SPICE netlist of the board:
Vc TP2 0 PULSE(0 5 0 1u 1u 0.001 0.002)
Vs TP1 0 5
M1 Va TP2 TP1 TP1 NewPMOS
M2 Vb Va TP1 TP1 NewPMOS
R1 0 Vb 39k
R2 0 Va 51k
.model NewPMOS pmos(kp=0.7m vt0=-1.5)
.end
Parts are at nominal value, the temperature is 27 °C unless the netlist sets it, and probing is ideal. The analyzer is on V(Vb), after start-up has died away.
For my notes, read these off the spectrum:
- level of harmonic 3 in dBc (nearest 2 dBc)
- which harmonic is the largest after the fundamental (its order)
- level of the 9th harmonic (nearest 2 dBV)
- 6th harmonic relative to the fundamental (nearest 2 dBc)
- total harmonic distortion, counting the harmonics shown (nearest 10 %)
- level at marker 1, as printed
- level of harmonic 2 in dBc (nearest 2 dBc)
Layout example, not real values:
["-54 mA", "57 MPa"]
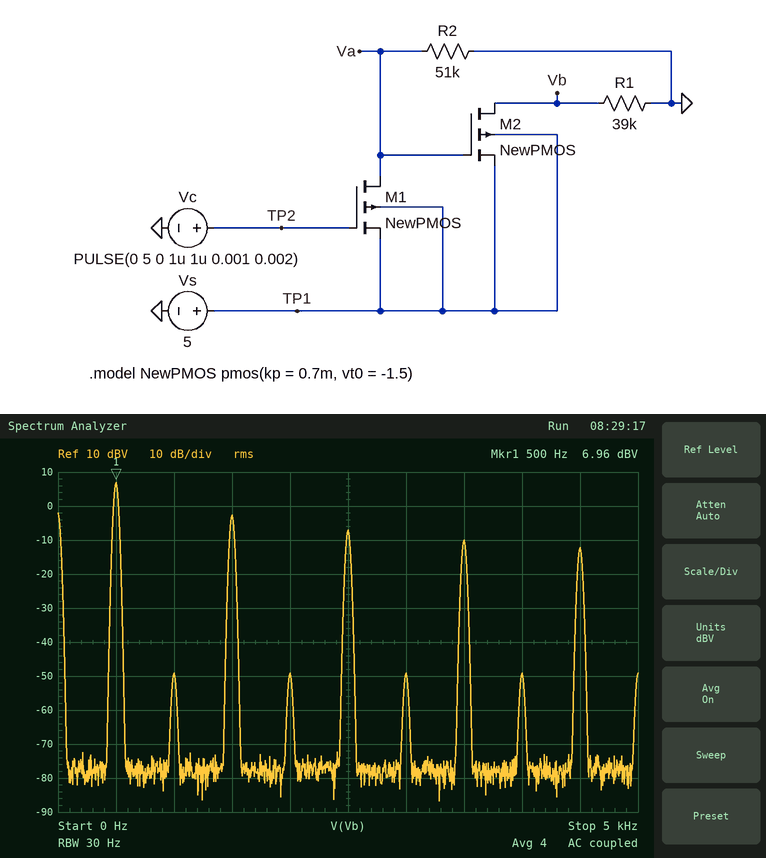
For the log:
["-10 dBc", "3", "-12 dBV", "-56 dBc", "40 %", "6.96 dBV", "-56 dBc"]
